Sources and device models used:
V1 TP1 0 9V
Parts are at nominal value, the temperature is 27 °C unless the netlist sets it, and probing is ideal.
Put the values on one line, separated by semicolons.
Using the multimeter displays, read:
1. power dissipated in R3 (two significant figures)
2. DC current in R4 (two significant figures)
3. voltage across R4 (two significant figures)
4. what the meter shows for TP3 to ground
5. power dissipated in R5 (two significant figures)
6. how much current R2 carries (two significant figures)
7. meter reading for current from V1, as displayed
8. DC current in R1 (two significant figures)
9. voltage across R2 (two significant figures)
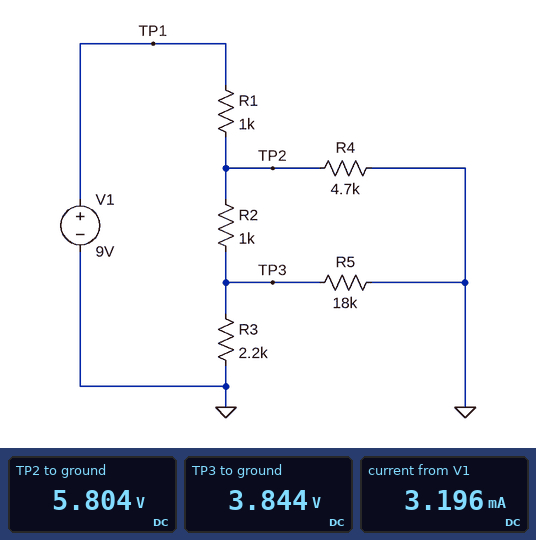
6.7 mW; 1.2 mA; 5.8 V; 3.844 V; 820 µW; 2.0 mA; 3.196 mA; 3.2 mA; 2.0 V
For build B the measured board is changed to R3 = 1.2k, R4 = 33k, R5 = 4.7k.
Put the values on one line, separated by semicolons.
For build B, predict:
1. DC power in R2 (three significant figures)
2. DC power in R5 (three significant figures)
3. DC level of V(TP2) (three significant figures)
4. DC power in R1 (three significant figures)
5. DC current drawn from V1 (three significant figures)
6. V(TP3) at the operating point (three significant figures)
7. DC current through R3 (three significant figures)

8.91 mW; 1.73 mW; 5.84 V; 10.0 mW; 3.16 mA; 2.85 V; 2.38 mA
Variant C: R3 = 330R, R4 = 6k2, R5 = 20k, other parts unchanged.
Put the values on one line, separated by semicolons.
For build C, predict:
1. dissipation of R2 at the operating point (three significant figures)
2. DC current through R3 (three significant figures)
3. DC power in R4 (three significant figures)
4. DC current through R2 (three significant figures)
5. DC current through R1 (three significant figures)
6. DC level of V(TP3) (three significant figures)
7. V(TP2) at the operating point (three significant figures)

12.6 mW; 3.49 mA; 3.56 mW; 3.55 mA; 4.30 mA; 1.15 V; 4.70 V
